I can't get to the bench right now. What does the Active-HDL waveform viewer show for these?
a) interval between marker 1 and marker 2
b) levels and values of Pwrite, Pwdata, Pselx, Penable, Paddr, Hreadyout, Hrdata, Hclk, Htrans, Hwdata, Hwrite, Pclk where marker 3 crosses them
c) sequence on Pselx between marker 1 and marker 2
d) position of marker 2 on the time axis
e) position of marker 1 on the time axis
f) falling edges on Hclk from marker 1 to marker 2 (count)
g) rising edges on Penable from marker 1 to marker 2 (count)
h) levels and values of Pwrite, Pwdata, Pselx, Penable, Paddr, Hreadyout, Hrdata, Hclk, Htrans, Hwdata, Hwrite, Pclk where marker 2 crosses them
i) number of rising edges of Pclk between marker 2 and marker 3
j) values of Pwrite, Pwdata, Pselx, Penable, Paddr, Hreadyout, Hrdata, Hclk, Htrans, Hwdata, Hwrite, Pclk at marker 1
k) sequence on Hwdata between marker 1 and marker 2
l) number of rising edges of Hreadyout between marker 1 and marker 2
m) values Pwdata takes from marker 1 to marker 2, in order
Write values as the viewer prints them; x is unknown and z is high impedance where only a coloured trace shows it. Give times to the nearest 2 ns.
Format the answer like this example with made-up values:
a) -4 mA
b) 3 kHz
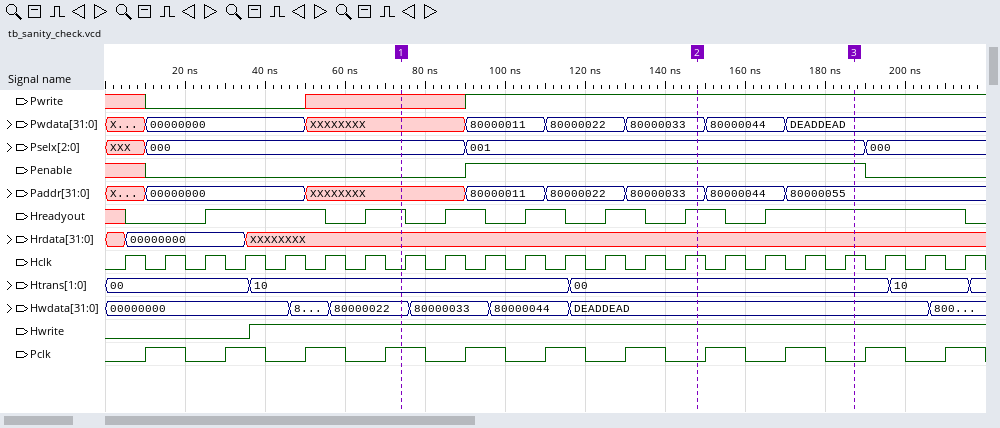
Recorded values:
a) 74 ns
b) Pwrite=1, Pwdata=DEADDEAD, Pselx=001, Penable=1, Paddr=80000055, Hreadyout=1, Hrdata=XXXXXXXX, Hclk=1, Htrans=00, Hwdata=DEADDEAD, Hwrite=1, Pclk=0
c) 000, 001
d) 148 ns
e) 74 ns
f) 7
g) 1
h) Pwrite=1, Pwdata=80000033, Pselx=001, Penable=1, Paddr=80000033, Hreadyout=1, Hrdata=XXXXXXXX, Hclk=1, Htrans=00, Hwdata=DEADDEAD, Hwrite=1, Pclk=0
i) 2
j) Pwrite=x, Pwdata=XXXXXXXX, Pselx=000, Penable=0, Paddr=XXXXXXXX, Hreadyout=1, Hrdata=XXXXXXXX, Hclk=0, Htrans=10, Hwdata=80000022, Hwrite=1, Pclk=1
k) 80000022, 80000033, 80000044, DEADDEAD
l) 4
m) XXXXXXXX, 80000011, 80000022, 80000033
